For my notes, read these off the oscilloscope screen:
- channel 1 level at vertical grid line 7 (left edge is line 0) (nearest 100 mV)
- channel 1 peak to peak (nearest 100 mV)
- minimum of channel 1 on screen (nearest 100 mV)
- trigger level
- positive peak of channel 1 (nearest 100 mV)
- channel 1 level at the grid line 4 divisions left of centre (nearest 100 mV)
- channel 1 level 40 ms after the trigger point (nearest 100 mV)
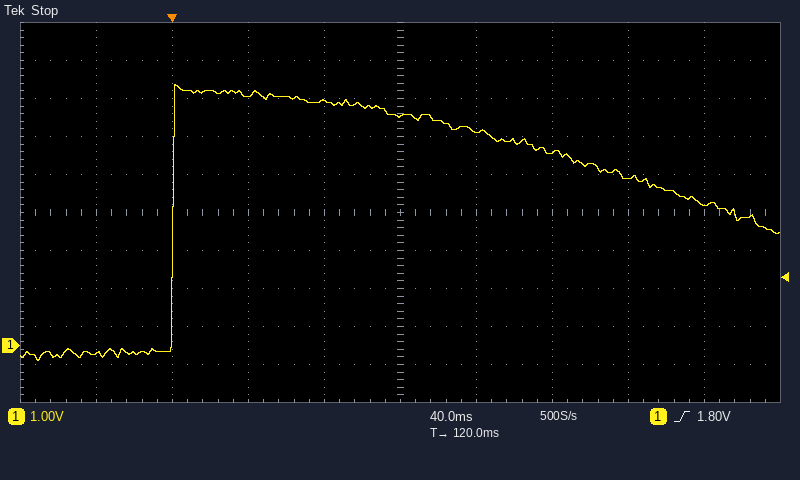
5.1 V
7.3 V
-400 mV
1.80 V
6.9 V
-200 mV
6.6 V
